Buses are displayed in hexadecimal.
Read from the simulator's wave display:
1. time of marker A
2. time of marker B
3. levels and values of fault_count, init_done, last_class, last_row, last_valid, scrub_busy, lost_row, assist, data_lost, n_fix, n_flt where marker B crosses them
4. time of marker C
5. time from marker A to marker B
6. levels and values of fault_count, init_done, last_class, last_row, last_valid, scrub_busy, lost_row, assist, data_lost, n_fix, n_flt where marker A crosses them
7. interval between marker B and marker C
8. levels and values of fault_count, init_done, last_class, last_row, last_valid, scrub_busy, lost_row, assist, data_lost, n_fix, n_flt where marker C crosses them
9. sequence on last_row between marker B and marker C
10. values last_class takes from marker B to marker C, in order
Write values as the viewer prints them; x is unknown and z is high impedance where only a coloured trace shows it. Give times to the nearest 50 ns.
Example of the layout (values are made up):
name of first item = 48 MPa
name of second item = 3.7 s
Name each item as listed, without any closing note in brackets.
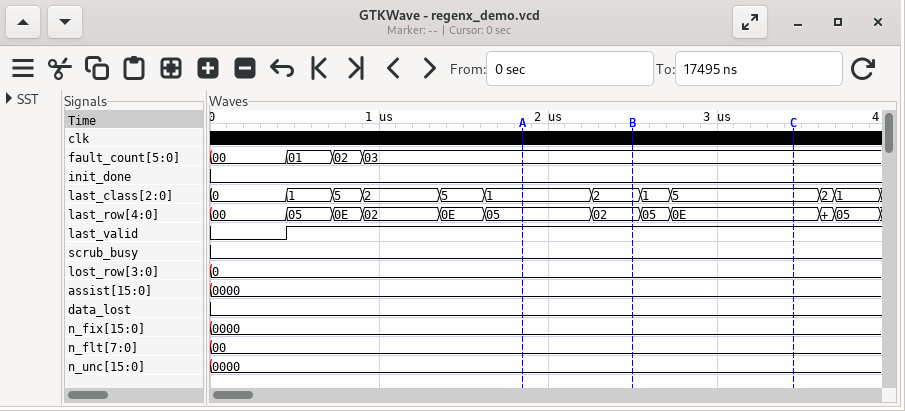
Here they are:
time of marker A = 1850 ns
time of marker B = 2500 ns
levels and values of fault_count, init_done, last_class, last_row, last_valid, scrub_busy, lost_row, assist, data_lost, n_fix, n_flt where marker B crosses them = fault_count=03, init_done=0, last_class=2, last_row=02, last_valid=1, scrub_busy=0, lost_row=0, assist=0000, data_lost=0, n_fix=0000, n_flt=00
time of marker C = 3450 ns
time from marker A to marker B = 650 ns
levels and values of fault_count, init_done, last_class, last_row, last_valid, scrub_busy, lost_row, assist, data_lost, n_fix, n_flt where marker A crosses them = fault_count=03, init_done=0, last_class=1, last_row=05, last_valid=1, scrub_busy=0, lost_row=0, assist=0000, data_lost=0, n_fix=0000, n_flt=00
interval between marker B and marker C = 950 ns
levels and values of fault_count, init_done, last_class, last_row, last_valid, scrub_busy, lost_row, assist, data_lost, n_fix, n_flt where marker C crosses them = fault_count=03, init_done=0, last_class=5, last_row=0E, last_valid=1, scrub_busy=0, lost_row=0, assist=0000, data_lost=0, n_fix=0000, n_flt=00
sequence on last_row between marker B and marker C = 02, 05, 0E
values last_class takes from marker B to marker C, in order = 2, 1, 5
